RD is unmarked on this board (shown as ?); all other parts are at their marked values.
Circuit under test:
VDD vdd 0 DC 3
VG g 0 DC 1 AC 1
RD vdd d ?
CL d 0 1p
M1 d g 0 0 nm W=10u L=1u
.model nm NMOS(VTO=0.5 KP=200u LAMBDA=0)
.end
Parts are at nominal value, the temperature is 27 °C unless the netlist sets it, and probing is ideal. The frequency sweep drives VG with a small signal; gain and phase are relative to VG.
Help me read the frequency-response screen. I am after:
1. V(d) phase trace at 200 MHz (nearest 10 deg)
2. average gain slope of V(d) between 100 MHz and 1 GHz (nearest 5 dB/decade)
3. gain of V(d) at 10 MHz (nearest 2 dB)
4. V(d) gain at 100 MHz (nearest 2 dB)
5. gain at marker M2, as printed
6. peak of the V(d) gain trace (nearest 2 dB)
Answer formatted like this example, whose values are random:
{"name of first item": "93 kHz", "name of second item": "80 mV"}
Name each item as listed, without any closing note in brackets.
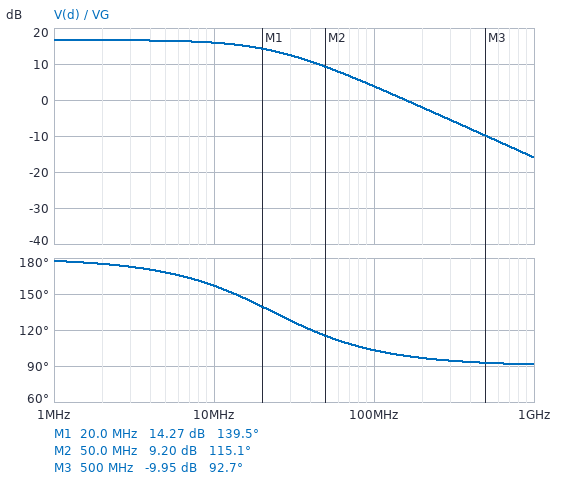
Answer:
{"V(d) phase trace at 200 MHz": "100 deg", "average gain slope of V(d) between 100 MHz and 1 GHz": "-20 dB/decade", "gain of V(d) at 10 MHz": "16 dB", "V(d) gain at 100 MHz": "4 dB", "gain at marker M2, as printed": "9.20 dB", "peak of the V(d) gain trace": "16 dB"}
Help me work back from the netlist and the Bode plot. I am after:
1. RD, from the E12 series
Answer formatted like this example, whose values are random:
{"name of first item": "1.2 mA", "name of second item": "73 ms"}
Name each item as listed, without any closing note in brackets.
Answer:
{"RD, from the E12 series": "6.8 kΩ"}
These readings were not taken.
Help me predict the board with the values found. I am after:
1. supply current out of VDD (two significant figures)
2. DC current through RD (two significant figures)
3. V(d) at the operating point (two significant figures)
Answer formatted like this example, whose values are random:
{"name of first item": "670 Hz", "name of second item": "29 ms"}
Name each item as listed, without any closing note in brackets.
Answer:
{"supply current out of VDD": "250 µA", "DC current through RD": "250 µA", "V(d) at the operating point": "1.3 V"}
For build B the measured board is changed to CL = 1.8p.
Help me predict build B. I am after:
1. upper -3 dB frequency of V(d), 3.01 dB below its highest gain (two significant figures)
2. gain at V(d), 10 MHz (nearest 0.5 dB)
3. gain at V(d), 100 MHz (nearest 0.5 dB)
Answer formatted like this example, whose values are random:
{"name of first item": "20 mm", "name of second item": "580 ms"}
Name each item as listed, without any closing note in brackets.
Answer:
{"upper -3 dB frequency of V(d), 3.01 dB below its highest gain": "13 MHz", "gain at V(d), 10 MHz": "14.5 dB", "gain at V(d), 100 MHz": "-1.0 dB"}
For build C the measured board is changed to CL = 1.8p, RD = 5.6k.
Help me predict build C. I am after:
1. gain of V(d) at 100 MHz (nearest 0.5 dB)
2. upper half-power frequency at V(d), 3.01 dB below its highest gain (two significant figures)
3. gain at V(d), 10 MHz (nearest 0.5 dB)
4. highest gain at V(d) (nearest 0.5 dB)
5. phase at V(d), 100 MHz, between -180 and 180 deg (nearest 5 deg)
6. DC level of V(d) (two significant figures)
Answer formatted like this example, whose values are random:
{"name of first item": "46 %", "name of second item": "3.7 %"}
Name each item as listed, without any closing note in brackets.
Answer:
{"gain of V(d) at 100 MHz": "-1.0 dB", "upper half-power frequency at V(d), 3.01 dB below its highest gain": "16 MHz", "gain at V(d), 10 MHz": "13.5 dB", "highest gain at V(d)": "15.0 dB", "phase at V(d), 100 MHz, between -180 and 180 deg": "100 deg", "DC level of V(d)": "1.6 V"}
